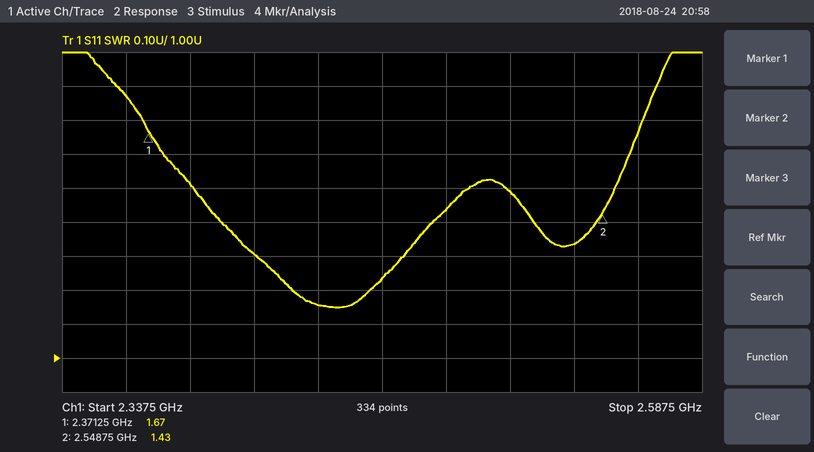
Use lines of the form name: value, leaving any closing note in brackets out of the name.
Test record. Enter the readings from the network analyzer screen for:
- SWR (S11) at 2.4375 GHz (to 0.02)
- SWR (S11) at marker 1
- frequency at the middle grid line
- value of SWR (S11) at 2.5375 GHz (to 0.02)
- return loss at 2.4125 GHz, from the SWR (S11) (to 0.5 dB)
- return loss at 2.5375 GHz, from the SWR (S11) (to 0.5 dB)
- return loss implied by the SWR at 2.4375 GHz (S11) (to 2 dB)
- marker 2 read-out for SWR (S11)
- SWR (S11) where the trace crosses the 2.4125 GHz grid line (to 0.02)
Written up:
SWR (S11) at 2.4375 GHz: 1.16
SWR (S11) at marker 1: 1.67
frequency at the middle grid line: 2.4625 GHz
value of SWR (S11) at 2.5375 GHz: 1.34
return loss at 2.4125 GHz, from the SWR (S11): 17.5 dB
return loss at 2.5375 GHz, from the SWR (S11): 17.0 dB
return loss implied by the SWR at 2.4375 GHz (S11): 22 dB
marker 2 read-out for SWR: 1.43
SWR (S11) where the trace crosses the 2.4125 GHz grid line: 1.30
